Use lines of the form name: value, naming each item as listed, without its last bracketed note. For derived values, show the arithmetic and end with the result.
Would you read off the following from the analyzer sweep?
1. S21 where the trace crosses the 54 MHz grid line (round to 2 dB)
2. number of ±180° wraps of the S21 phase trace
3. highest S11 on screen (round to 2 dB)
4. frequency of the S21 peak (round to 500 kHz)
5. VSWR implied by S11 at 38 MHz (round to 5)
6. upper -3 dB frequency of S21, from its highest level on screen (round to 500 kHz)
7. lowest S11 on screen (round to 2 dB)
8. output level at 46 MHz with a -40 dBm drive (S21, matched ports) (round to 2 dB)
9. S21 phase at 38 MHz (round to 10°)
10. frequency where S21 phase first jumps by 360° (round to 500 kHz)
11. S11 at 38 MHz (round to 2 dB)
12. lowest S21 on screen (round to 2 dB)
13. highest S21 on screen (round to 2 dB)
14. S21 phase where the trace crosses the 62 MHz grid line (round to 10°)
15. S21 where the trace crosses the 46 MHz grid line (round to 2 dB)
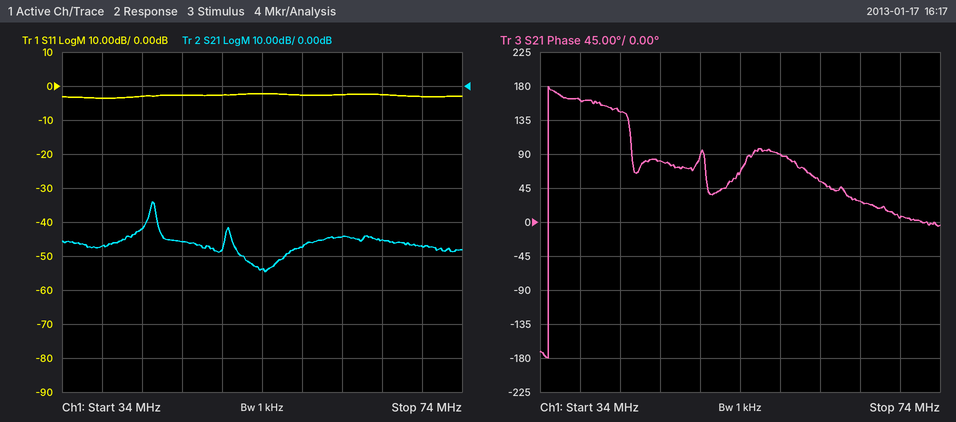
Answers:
S21 where the trace crosses the 54 MHz grid line: -54 dB
number of ±180° wraps of the S21 phase trace: 1
highest S11 on screen: -2 dB
frequency of the S21 peak: 43.0 MHz
VSWR implied by S11 at 38 MHz: |Γ| = 10^(-4/20) = 0.6310; VSWR = (1 + 0.6310)/(1 − 0.6310) ≈ 4.42, so 5 to the nearest 5
upper -3 dB frequency of S21, from its highest level on screen: 43.5 MHz
lowest S11 on screen: -4 dB
output level at 46 MHz with a -40 dBm drive (S21, matched ports): -40 dBm + (-46 dB) = -86 dBm
S21 phase at 38 MHz: 160°
frequency where S21 phase first jumps by 360°: 35.0 MHz
S11 at 38 MHz: -4 dB
lowest S21 on screen: -54 dB
highest S21 on screen: -34 dB
S21 phase where the trace crosses the 62 MHz grid line: 50°
S21 where the trace crosses the 46 MHz grid line: -46 dB
